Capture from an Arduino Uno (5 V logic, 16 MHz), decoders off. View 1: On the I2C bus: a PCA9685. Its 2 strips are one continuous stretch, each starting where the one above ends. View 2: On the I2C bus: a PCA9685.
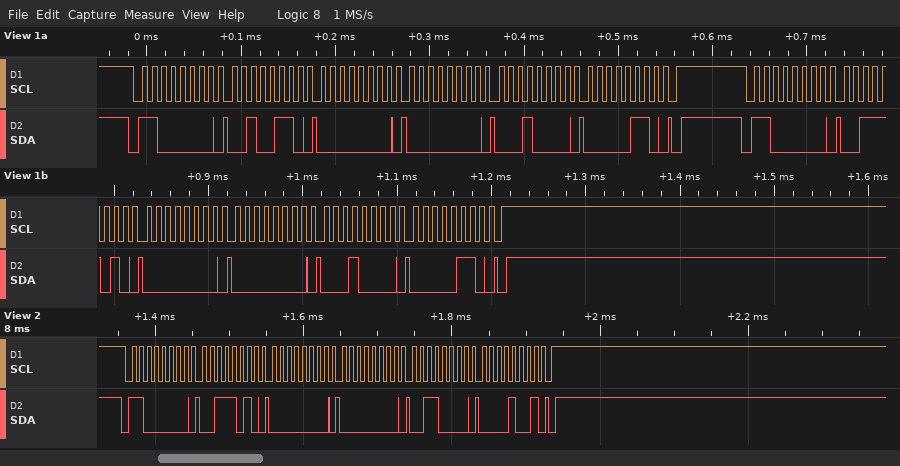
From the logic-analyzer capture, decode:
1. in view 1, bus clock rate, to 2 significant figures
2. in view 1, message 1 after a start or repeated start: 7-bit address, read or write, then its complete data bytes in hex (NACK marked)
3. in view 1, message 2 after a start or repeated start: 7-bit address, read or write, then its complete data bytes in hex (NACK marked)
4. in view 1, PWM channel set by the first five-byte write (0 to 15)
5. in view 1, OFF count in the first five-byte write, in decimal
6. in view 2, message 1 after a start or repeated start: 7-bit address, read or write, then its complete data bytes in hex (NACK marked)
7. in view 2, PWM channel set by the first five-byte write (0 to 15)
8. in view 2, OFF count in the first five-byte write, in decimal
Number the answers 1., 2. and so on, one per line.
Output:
1. 100 kHz
2. 0x60 write: 26 00 00 10 06
3. 0x60 write: 3A 00 00 10 06
4. 8
5. 1552
6. 0x60 write: 3A 00 00 30 09
7. 13
8. 2352
